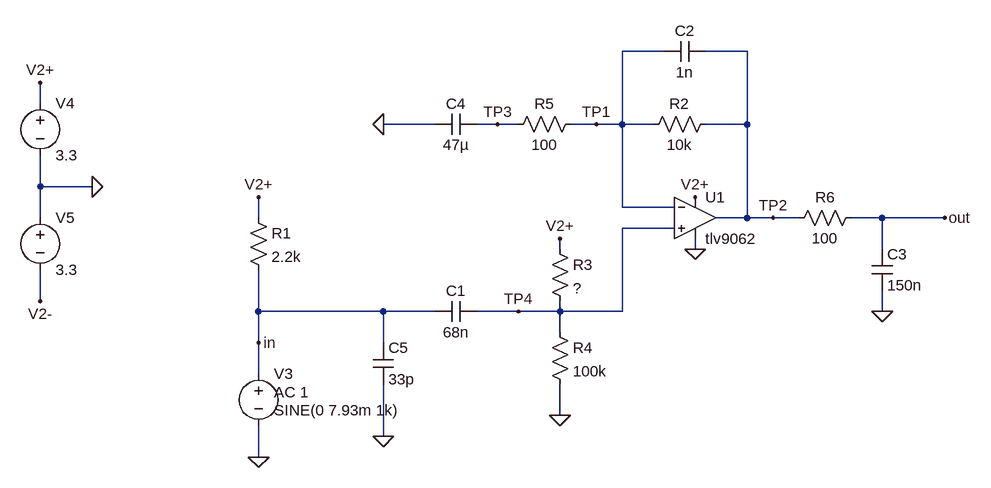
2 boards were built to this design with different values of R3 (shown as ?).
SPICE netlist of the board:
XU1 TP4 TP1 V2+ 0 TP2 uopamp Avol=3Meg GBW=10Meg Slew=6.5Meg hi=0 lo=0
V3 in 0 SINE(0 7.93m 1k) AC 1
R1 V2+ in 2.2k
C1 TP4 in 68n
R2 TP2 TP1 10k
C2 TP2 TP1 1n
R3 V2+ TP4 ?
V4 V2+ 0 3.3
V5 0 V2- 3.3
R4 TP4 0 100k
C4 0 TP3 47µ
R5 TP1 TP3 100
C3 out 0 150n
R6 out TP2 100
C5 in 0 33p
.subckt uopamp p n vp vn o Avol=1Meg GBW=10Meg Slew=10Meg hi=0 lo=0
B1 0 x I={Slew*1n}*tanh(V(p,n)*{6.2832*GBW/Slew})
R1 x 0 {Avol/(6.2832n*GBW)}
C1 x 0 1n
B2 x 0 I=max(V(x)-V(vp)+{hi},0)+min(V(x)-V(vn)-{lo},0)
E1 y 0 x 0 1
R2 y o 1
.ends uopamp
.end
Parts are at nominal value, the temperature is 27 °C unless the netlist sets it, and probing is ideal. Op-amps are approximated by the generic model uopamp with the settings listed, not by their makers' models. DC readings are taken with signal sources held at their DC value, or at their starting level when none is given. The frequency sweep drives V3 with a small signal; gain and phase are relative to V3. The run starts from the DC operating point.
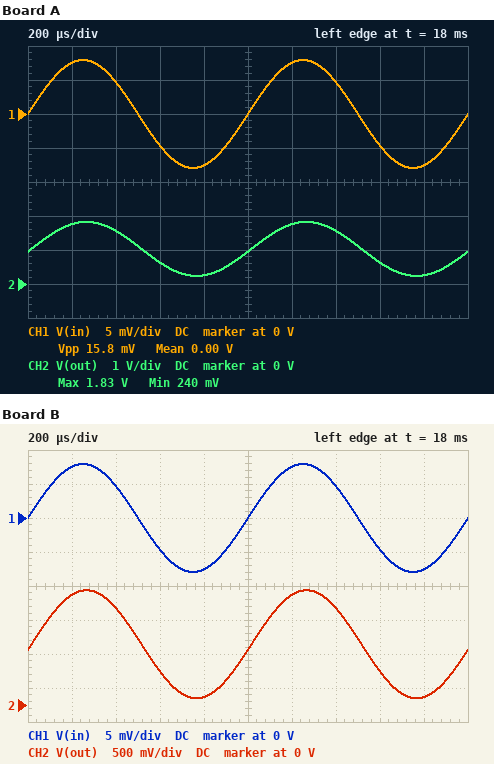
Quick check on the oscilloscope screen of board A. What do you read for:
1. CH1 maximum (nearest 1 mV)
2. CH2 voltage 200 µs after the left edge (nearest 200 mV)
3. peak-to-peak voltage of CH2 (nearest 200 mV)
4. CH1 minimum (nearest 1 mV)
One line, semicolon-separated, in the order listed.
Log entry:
8 mV; 1.8 V; 1.6 V; -8 mV
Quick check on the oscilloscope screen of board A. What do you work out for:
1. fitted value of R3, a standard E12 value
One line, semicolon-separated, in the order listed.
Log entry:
220 kΩ
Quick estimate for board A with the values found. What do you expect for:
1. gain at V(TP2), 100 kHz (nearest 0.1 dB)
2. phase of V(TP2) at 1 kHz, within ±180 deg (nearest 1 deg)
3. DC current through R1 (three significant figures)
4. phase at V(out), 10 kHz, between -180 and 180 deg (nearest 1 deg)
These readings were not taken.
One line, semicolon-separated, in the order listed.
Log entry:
22.8 dB; 0 deg; 1.50 mA; -79 deg
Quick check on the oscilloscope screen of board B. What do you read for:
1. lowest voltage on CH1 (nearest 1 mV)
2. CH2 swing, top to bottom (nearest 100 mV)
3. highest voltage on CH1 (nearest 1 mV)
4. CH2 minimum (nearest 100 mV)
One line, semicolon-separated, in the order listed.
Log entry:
-8 mV; 1.6 V; 8 mV; 100 mV
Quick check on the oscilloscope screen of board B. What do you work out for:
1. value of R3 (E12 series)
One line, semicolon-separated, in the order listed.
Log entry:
270 kΩ
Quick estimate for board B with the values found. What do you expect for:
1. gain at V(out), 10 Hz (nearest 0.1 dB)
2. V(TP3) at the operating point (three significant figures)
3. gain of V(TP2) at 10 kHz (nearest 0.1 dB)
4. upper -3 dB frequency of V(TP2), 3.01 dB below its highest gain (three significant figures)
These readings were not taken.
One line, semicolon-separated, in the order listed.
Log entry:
18.6 dB; 892 mV; 38.2 dB; 13.8 kHz
